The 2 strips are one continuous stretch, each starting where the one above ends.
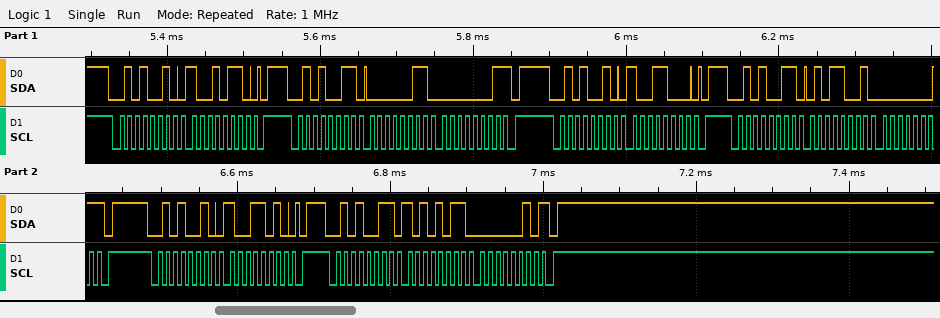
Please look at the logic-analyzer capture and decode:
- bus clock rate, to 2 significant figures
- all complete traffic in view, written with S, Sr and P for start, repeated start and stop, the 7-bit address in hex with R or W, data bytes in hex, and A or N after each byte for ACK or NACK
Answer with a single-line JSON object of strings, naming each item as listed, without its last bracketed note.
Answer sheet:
{"bus clock rate, to 2 significant figures": "100 kHz", "all complete traffic in view, written with S, Sr and P for start, repeated start and stop, the 7-bit address in hex with R or W, data bytes in hex, and A or N after each byte for ACK or NACK": "S 29W A 96 A P S 29R A 03 A 01 N P S 29W A 98 A P S 29R A 59 A 01 N P S 29W A 9A A P S 29R A AB A 02 N P"}
